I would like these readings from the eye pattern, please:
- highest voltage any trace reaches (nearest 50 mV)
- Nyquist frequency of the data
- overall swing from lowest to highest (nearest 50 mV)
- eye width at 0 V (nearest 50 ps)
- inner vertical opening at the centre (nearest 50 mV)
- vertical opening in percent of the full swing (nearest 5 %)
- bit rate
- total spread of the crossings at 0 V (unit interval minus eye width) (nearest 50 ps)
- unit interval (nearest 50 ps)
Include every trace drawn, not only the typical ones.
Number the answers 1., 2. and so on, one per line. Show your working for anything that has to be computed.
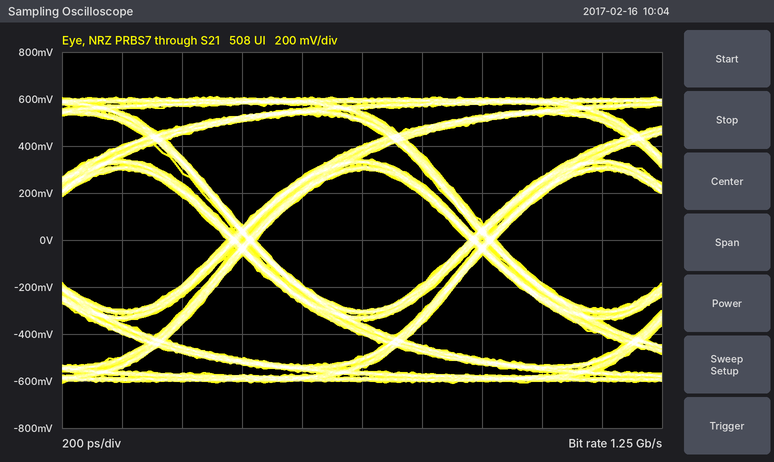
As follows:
1. 600 mV
2. 625 MHz
3. 1.20 V
4. 700 ps
5. 600 mV
6. 600 mV / 1.20 V ≈ 50 %
7. 1.25 Gb/s
8. 100 ps
9. 800 ps
